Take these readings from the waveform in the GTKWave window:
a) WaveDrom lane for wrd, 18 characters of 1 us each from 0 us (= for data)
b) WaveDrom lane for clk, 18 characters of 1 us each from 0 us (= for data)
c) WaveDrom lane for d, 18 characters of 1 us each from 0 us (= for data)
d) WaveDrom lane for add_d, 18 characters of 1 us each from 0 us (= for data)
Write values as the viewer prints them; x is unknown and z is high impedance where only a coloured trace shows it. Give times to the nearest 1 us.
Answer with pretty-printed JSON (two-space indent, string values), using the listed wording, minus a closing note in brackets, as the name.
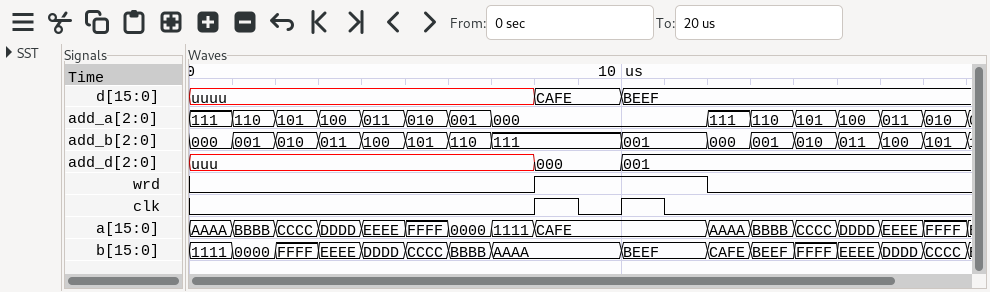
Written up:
{
  "WaveDrom lane for wrd, 18 characters of 1 us each from 0 us": "{name: 'wrd', wave: '0.......1...0.....'}",
  "WaveDrom lane for clk, 18 characters of 1 us each from 0 us": "{name: 'clk', wave: '0.......1010......'}",
  "WaveDrom lane for d, 18 characters of 1 us each from 0 us": "{name: 'd', wave: 'x.......=.=.......', data: 'CAFE BEEF'}",
  "WaveDrom lane for add_d, 18 characters of 1 us each from 0 us": "{name: 'add_d', wave: 'x.......=.=.......', data: '000 001'}"
}
